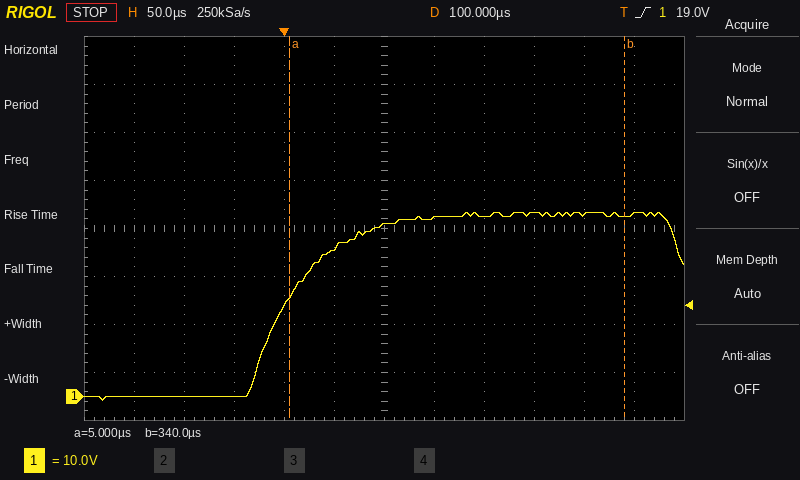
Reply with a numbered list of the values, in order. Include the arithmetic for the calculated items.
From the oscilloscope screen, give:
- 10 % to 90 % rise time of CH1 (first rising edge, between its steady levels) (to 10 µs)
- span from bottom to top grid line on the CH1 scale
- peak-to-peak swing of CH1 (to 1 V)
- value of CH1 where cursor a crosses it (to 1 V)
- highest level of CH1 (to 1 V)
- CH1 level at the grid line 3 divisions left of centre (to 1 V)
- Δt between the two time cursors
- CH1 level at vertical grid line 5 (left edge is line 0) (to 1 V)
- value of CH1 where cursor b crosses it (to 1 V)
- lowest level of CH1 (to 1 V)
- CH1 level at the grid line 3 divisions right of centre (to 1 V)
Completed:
1. 100 µs
2. 80 V
3. 38 V − (-1 V) = 39 V
4. 21 V
5. 38 V
6. 0 V
7. 340 µs − (5 µs) = 335 µs
8. 31 V
9. 38 V
10. -1 V
11. 38 V
